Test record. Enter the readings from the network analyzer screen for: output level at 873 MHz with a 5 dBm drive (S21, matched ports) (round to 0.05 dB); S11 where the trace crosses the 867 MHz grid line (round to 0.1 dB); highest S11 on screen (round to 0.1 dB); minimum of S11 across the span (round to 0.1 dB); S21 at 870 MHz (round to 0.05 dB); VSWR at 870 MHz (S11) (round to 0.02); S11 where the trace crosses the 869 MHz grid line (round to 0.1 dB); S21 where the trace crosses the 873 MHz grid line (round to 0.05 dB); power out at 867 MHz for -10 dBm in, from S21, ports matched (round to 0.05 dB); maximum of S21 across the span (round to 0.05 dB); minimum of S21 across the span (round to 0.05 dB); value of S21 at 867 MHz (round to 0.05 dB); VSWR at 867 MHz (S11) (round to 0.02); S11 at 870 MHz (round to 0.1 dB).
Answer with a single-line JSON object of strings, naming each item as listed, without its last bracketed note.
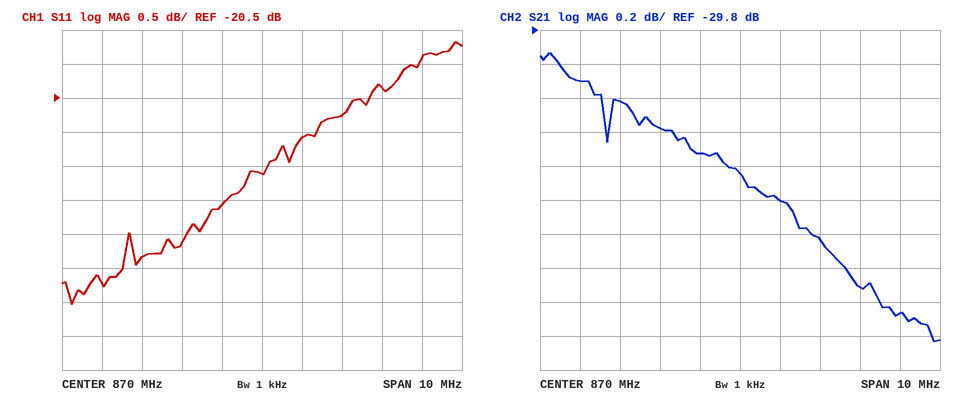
{"output level at 873 MHz with a 5 dBm drive (S21, matched ports)": "-26.30 dBm", "S11 where the trace crosses the 867 MHz grid line": "-22.8 dB", "highest S11 on screen": "-19.7 dB", "minimum of S11 across the span": "-23.5 dB", "S21 at 870 MHz": "-30.65 dB", "VSWR at 870 MHz (S11)": "1.18", "S11 where the trace crosses the 869 MHz grid line": "-22.1 dB", "S21 where the trace crosses the 873 MHz grid line": "-31.30 dB", "power out at 867 MHz for -10 dBm in, from S21, ports matched": "-40.20 dBm", "maximum of S21 across the span": "-29.95 dB", "minimum of S21 across the span": "-31.65 dB", "value of S21 at 867 MHz": "-30.20 dB", "VSWR at 867 MHz (S11)": "1.16", "S11 at 870 MHz": "-21.6 dB"}
